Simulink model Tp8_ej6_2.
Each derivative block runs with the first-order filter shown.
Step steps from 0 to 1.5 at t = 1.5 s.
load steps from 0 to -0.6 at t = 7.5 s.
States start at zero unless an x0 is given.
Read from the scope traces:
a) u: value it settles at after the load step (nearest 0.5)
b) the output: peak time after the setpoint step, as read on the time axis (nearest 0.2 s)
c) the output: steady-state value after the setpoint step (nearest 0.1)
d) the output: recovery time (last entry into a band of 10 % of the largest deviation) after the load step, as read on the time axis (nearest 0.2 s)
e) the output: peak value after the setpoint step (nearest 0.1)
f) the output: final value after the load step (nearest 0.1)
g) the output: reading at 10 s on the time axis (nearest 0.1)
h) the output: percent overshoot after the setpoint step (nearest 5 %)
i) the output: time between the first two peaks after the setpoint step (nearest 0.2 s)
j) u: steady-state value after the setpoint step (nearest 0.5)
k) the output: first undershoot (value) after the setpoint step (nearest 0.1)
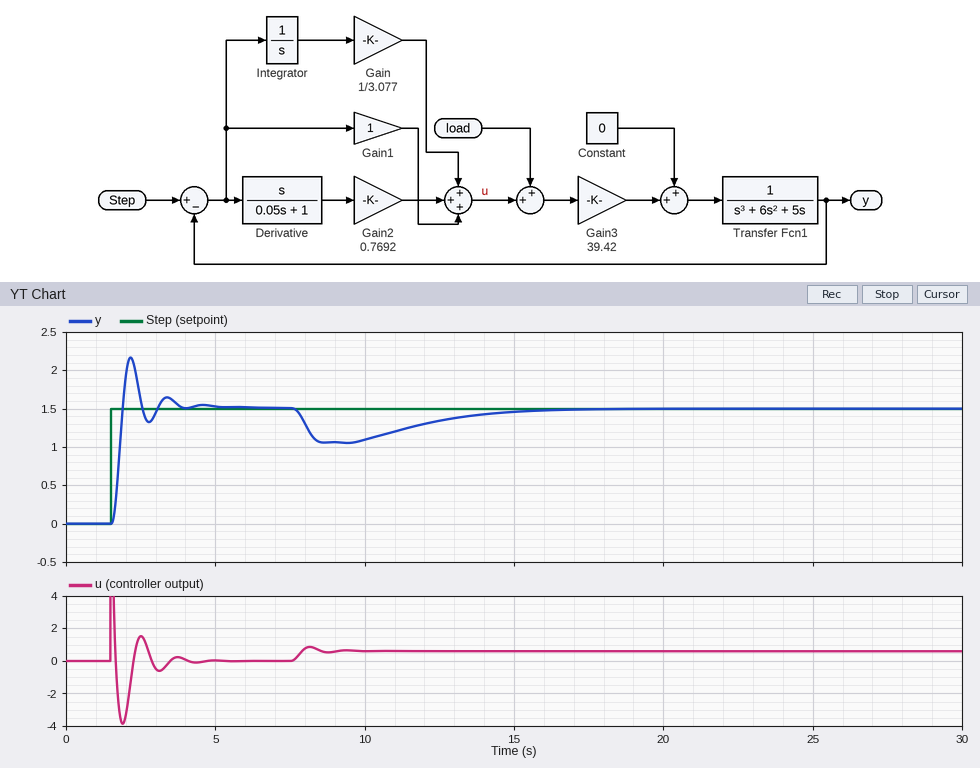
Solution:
0.5
2.2 s
1.5
14.8 s
2.2
1.5
1.1
45 %
1.2 s
0.0
1.3
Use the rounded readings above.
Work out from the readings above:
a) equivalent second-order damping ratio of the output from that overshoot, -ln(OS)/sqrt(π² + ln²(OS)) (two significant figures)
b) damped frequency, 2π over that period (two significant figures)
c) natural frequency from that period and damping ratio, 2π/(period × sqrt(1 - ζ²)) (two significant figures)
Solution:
0.25
5.2 rad/s
5.4 rad/s
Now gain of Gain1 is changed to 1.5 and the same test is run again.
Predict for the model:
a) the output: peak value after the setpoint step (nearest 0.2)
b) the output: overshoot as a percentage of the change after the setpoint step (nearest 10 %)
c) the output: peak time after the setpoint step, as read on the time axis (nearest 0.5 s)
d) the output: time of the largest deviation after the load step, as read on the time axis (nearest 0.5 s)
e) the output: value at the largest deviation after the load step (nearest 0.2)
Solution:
2.4
60 %
2.0 s
8.5 s
1.2
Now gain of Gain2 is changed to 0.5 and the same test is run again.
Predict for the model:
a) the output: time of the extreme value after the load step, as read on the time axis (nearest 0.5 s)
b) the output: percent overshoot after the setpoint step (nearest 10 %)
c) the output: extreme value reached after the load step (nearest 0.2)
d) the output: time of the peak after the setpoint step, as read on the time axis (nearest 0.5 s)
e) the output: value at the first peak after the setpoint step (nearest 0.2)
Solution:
8.5 s
50 %
1.0
2.5 s
2.2
